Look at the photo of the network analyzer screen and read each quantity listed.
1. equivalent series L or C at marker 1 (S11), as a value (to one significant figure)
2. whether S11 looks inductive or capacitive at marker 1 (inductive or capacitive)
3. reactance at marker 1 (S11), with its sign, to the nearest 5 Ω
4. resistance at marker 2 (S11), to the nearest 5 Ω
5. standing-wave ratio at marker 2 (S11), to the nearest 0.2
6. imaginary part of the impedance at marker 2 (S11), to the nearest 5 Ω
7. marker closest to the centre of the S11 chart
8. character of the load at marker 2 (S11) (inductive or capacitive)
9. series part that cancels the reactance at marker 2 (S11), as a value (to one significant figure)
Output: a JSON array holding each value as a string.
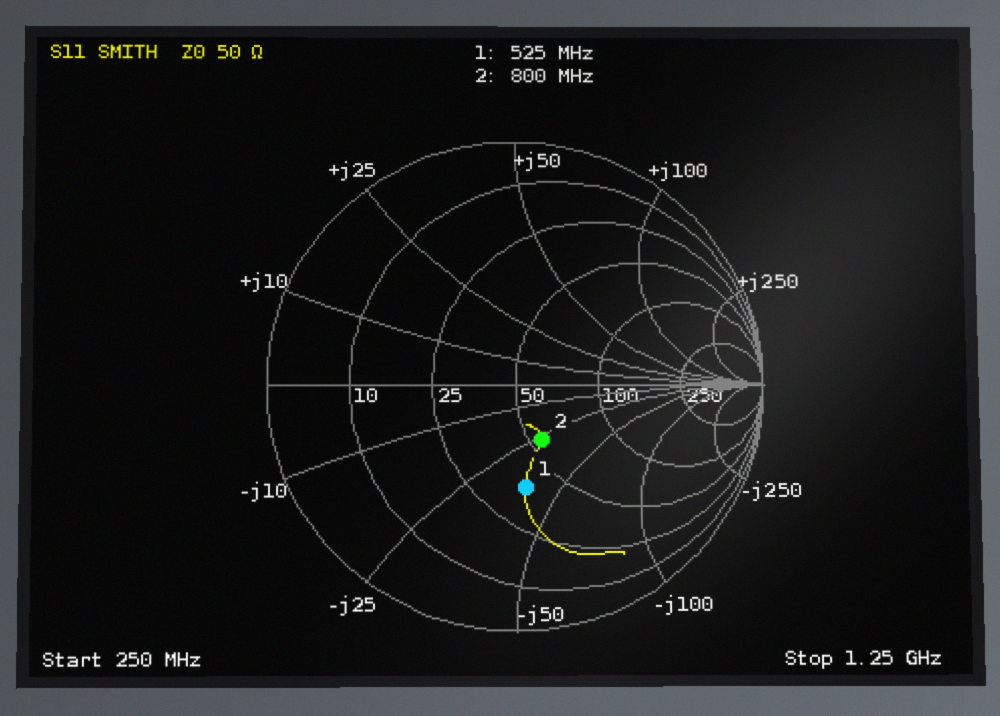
["8 pF", "capacitive", "-40 Ω", "55 Ω", "1.6", "-25 Ω", "marker 2", "capacitive", "5 nH"]
